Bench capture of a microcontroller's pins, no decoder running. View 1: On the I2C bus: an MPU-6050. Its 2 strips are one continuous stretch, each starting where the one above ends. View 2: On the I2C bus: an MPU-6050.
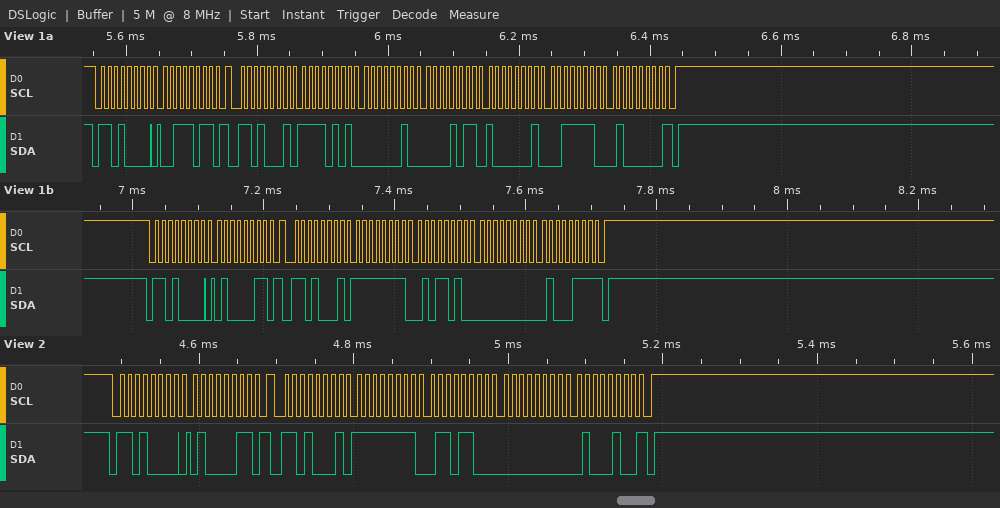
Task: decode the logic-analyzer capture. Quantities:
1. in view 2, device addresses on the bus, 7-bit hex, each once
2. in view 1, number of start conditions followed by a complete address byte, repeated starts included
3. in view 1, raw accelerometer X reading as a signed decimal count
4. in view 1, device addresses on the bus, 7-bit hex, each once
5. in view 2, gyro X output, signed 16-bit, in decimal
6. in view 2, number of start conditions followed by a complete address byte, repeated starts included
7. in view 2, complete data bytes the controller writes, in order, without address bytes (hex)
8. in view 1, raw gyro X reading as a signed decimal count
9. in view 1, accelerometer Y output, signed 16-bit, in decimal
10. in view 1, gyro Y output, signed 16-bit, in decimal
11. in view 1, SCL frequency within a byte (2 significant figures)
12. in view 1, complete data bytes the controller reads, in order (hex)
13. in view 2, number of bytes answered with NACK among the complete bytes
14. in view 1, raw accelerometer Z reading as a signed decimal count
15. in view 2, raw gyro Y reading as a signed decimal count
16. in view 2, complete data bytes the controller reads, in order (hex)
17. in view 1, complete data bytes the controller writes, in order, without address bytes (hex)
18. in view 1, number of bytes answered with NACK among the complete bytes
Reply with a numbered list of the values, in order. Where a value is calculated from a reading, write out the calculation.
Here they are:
1. 0x68
2. 4
3. 0xF502 = -2814
4. 0x68
5. 0xFF6C = -148
6. 2
7. 43
8. 0xFF5A = -166
9. 0x0B81 = 2945
10. 0x0047 = 71
11. 100 kHz
12. F5 02 0B 81 3E 40 FF 5A 00 47
13. 1
14. 0x3E40 = 15936
15. 0x0044 = 68
16. FF 6C 00 44
17. 3B 43
18. 2
